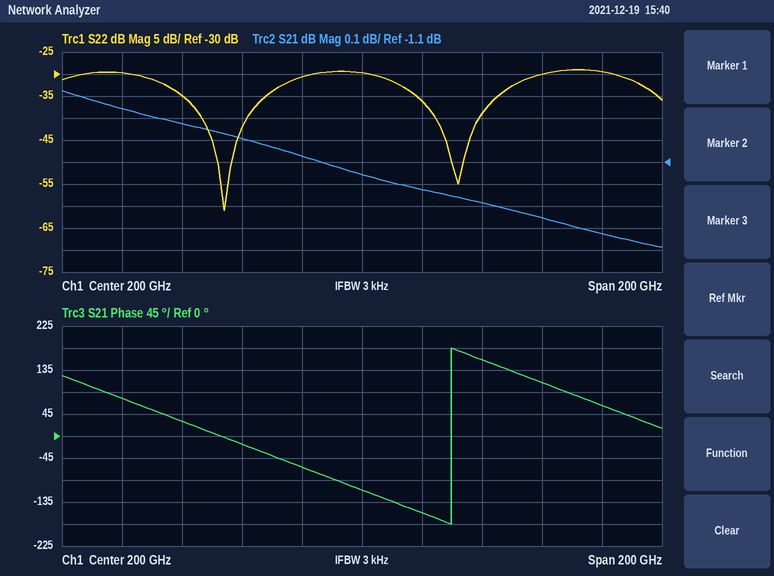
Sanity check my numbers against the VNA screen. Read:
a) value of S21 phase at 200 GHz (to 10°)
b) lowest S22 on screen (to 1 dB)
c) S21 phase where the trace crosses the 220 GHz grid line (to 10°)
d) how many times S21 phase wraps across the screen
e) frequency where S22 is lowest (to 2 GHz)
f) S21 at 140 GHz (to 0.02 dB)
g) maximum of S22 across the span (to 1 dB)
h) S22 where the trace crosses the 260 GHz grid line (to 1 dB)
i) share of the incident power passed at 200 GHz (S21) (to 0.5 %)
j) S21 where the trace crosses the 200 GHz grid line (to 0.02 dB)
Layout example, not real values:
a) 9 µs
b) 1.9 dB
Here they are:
a) -110°
b) -61 dB
c) -160°
d) 1
e) 154 GHz
f) -0.92 dB
g) -29 dB
h) -30 dB
i) 76.5 %
j) -1.16 dB
